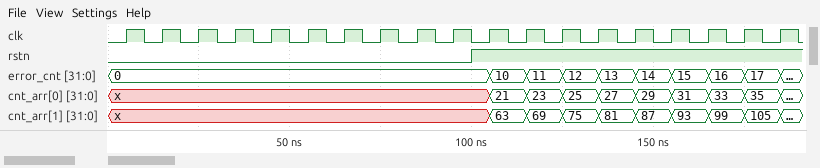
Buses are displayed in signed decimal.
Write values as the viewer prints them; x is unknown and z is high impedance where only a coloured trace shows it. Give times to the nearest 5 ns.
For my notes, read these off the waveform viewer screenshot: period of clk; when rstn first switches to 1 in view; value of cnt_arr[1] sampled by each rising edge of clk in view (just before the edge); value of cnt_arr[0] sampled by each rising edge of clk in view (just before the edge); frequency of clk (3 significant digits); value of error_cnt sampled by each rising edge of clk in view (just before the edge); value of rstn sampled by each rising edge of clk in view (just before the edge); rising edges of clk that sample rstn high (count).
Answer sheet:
10 ns
100 ns
x, x, x, x, x, x, x, x, x, x, x, 63, 69, 75, 81, 87, 93, 99, 105
x, x, x, x, x, x, x, x, x, x, x, 21, 23, 25, 27, 29, 31, 33, 35
100 MHz
0, 0, 0, 0, 0, 0, 0, 0, 0, 0, 0, 10, 11, 12, 13, 14, 15, 16, 17
0 0 0 0 0 0 0 0 0 0 1 1 1 1 1 1 1 1 1
9
